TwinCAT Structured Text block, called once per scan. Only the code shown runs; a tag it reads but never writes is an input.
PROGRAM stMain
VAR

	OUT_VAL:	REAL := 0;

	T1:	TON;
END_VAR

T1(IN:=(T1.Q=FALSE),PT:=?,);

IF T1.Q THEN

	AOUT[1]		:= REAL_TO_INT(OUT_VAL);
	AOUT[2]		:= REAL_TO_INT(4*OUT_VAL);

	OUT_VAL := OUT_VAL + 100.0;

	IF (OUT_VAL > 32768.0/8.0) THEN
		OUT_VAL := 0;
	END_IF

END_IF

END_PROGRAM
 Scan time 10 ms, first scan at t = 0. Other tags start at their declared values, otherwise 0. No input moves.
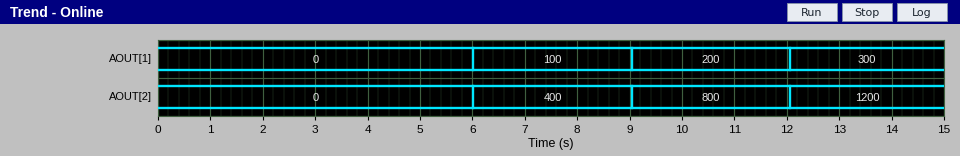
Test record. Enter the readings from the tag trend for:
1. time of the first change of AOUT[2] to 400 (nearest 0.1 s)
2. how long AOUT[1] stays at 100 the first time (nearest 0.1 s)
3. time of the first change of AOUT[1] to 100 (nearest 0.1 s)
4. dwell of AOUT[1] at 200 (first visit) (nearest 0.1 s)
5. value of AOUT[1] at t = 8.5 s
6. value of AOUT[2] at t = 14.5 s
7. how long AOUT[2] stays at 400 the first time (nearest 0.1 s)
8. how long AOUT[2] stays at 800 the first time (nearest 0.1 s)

6.0 s
3.0 s
6.0 s
3.0 s
100
1200
3.0 s
3.0 s
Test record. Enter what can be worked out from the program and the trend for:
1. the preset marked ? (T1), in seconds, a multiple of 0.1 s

3.0 s
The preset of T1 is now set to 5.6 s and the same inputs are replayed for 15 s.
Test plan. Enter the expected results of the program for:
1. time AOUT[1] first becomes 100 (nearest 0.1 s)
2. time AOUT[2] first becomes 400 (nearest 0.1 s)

11.2 s
11.2 s
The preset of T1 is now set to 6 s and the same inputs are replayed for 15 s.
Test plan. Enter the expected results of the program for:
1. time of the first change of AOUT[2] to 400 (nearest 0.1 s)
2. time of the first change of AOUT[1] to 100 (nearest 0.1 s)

12.0 s
12.0 s
